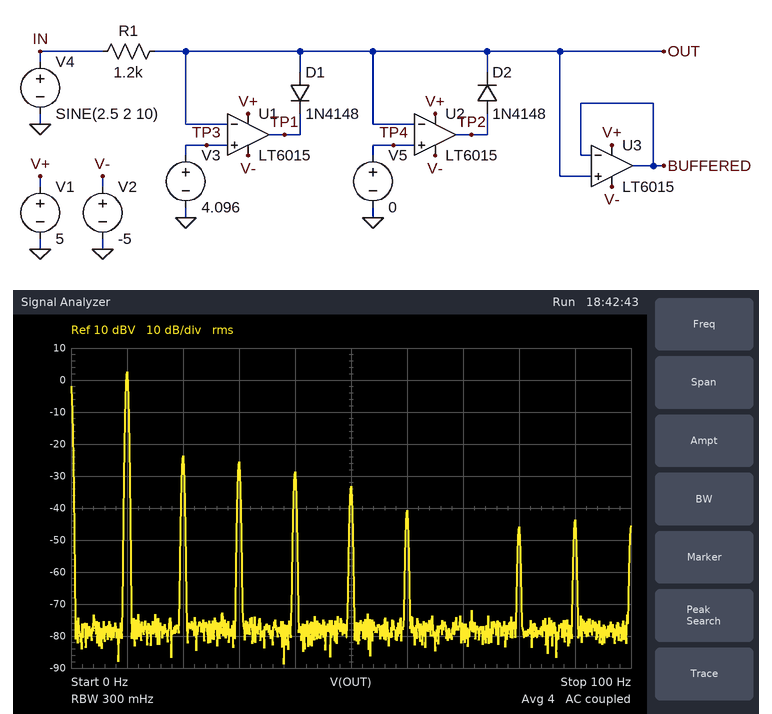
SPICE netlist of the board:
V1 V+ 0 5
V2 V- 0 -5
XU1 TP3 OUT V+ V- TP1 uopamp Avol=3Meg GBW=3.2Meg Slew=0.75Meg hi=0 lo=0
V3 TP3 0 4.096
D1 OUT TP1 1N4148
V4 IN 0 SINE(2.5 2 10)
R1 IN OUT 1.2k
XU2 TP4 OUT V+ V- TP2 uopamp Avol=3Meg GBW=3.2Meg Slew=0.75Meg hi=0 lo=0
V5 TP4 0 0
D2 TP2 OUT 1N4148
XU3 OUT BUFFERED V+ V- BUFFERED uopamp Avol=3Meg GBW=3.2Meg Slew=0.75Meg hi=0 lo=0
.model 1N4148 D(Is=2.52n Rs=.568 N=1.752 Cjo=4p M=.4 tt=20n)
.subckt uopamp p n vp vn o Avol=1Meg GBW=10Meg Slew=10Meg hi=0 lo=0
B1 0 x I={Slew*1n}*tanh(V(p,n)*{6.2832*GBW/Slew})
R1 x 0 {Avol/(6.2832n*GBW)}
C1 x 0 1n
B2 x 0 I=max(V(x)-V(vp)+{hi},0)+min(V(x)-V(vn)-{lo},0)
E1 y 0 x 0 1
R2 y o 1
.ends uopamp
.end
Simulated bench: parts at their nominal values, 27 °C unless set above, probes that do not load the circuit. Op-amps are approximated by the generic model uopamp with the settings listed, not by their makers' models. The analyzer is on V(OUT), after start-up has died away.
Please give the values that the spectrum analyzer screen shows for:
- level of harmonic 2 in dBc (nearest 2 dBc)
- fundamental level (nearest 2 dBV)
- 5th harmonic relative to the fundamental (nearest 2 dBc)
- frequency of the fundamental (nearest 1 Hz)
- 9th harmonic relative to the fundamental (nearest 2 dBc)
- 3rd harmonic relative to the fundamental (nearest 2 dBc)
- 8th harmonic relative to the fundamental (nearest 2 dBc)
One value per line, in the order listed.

-26 dBc
2 dBV
-36 dBc
10 Hz
-46 dBc
-28 dBc
-48 dBc
